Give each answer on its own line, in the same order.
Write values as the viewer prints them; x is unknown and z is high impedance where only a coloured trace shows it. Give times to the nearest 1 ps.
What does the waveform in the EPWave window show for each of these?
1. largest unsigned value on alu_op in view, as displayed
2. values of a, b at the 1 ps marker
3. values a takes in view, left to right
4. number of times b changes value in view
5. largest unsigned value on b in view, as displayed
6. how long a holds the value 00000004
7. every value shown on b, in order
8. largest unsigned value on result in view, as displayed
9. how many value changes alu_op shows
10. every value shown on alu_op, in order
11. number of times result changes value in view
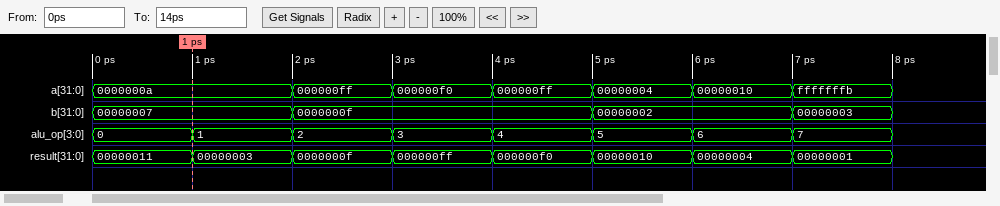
7
a=0000000a, b=00000007
0000000a, 000000ff, 000000f0, 000000ff, 00000004, 00000010, fffffffb
3
0000000f
1 ps
00000007, 0000000f, 00000002, 00000003
000000ff
7
0, 1, 2, 3, 4, 5, 6, 7
7
